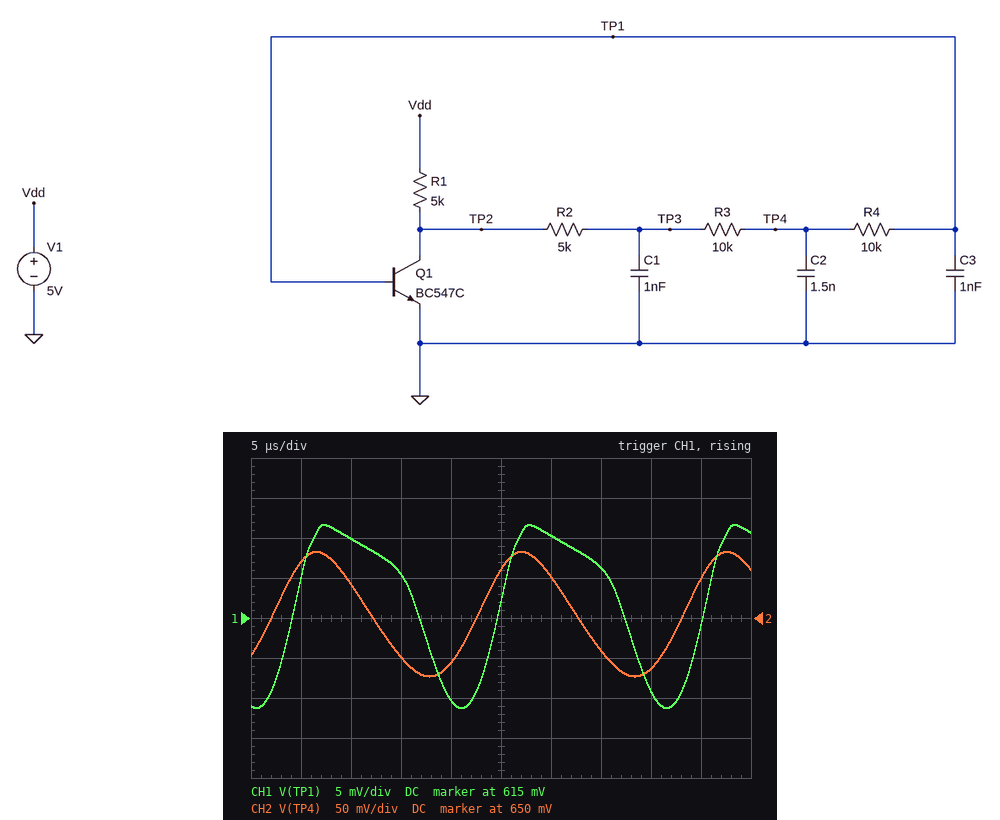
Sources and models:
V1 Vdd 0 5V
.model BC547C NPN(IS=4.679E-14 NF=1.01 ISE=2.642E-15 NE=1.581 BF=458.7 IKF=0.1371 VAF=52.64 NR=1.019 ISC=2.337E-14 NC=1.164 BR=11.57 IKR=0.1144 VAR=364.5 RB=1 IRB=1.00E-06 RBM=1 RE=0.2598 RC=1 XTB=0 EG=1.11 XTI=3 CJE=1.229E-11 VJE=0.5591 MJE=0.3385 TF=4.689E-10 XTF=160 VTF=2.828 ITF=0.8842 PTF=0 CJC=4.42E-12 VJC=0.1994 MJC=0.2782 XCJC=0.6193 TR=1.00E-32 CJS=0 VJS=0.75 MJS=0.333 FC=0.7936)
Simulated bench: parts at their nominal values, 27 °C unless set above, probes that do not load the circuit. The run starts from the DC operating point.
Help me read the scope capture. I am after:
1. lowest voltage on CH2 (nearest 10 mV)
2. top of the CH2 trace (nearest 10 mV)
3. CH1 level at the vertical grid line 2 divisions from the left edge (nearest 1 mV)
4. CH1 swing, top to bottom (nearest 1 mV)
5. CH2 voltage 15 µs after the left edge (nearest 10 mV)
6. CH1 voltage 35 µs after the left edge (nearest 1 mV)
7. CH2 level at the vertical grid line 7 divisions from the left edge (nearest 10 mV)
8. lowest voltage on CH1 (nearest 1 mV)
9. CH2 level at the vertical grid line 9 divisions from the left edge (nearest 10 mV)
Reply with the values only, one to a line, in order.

580 mV
730 mV
625 mV
23 mV
600 mV
621 mV
610 mV
604 mV
700 mV
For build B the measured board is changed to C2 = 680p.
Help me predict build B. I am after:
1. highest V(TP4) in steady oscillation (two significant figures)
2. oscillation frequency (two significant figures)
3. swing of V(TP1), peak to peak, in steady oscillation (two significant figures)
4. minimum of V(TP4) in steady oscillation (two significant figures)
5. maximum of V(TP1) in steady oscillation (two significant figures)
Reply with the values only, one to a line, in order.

760 mV
64 kHz
24 mV
560 mV
630 mV
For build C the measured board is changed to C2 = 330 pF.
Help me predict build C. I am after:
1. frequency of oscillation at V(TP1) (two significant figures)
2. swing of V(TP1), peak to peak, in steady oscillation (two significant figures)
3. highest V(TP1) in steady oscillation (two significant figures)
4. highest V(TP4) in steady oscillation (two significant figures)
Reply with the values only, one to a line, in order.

82 kHz
21 mV
630 mV
750 mV
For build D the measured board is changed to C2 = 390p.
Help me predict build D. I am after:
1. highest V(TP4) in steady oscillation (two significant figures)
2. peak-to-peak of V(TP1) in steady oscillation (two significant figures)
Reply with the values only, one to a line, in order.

750 mV
22 mV
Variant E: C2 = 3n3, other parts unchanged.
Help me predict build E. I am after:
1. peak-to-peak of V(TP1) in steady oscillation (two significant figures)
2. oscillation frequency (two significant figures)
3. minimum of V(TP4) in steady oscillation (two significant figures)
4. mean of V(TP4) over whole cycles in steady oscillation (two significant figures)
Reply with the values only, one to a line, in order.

19 mV
38 kHz
600 mV
640 mV
